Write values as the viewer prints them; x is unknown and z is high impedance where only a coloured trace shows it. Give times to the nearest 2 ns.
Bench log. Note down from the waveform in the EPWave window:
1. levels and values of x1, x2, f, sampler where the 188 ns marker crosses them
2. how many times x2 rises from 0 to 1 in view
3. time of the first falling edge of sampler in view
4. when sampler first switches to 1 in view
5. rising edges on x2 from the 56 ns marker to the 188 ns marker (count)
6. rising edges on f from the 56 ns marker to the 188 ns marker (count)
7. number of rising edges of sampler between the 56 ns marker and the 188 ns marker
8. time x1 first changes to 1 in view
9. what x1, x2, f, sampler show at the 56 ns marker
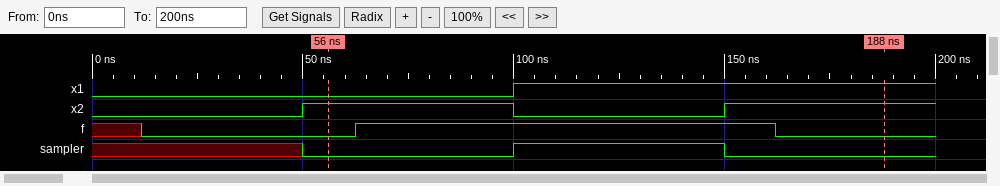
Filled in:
x1=1, x2=1, f=0, sampler=0
2
150 ns
100 ns
1
1
1
100 ns
x1=0, x2=1, f=0, sampler=0
